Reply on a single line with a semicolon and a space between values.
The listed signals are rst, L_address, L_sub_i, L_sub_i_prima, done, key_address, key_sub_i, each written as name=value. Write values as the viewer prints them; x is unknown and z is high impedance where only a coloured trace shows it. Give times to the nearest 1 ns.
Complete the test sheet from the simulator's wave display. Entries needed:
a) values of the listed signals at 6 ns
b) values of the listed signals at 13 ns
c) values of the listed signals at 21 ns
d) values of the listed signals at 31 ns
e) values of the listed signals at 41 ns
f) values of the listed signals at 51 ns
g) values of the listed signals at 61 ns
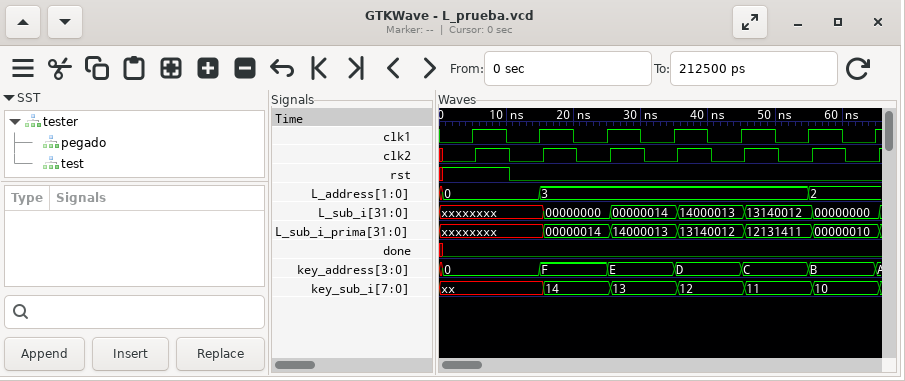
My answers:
rst=1, L_address=0, L_sub_i=xxxxxxxx, L_sub_i_prima=xxxxxxxx, done=0, key_address=0, key_sub_i=xx; rst=0, L_address=0, L_sub_i=xxxxxxxx, L_sub_i_prima=xxxxxxxx, done=0, key_address=0, key_sub_i=xx; rst=0, L_address=3, L_sub_i=00000000, L_sub_i_prima=00000014, done=0, key_address=F, key_sub_i=14; rst=0, L_address=3, L_sub_i=00000014, L_sub_i_prima=14000013, done=0, key_address=E, key_sub_i=13; rst=0, L_address=3, L_sub_i=14000013, L_sub_i_prima=13140012, done=0, key_address=D, key_sub_i=12; rst=0, L_address=3, L_sub_i=13140012, L_sub_i_prima=12131411, done=0, key_address=C, key_sub_i=11; rst=0, L_address=2, L_sub_i=00000000, L_sub_i_prima=00000010, done=0, key_address=B, key_sub_i=10
